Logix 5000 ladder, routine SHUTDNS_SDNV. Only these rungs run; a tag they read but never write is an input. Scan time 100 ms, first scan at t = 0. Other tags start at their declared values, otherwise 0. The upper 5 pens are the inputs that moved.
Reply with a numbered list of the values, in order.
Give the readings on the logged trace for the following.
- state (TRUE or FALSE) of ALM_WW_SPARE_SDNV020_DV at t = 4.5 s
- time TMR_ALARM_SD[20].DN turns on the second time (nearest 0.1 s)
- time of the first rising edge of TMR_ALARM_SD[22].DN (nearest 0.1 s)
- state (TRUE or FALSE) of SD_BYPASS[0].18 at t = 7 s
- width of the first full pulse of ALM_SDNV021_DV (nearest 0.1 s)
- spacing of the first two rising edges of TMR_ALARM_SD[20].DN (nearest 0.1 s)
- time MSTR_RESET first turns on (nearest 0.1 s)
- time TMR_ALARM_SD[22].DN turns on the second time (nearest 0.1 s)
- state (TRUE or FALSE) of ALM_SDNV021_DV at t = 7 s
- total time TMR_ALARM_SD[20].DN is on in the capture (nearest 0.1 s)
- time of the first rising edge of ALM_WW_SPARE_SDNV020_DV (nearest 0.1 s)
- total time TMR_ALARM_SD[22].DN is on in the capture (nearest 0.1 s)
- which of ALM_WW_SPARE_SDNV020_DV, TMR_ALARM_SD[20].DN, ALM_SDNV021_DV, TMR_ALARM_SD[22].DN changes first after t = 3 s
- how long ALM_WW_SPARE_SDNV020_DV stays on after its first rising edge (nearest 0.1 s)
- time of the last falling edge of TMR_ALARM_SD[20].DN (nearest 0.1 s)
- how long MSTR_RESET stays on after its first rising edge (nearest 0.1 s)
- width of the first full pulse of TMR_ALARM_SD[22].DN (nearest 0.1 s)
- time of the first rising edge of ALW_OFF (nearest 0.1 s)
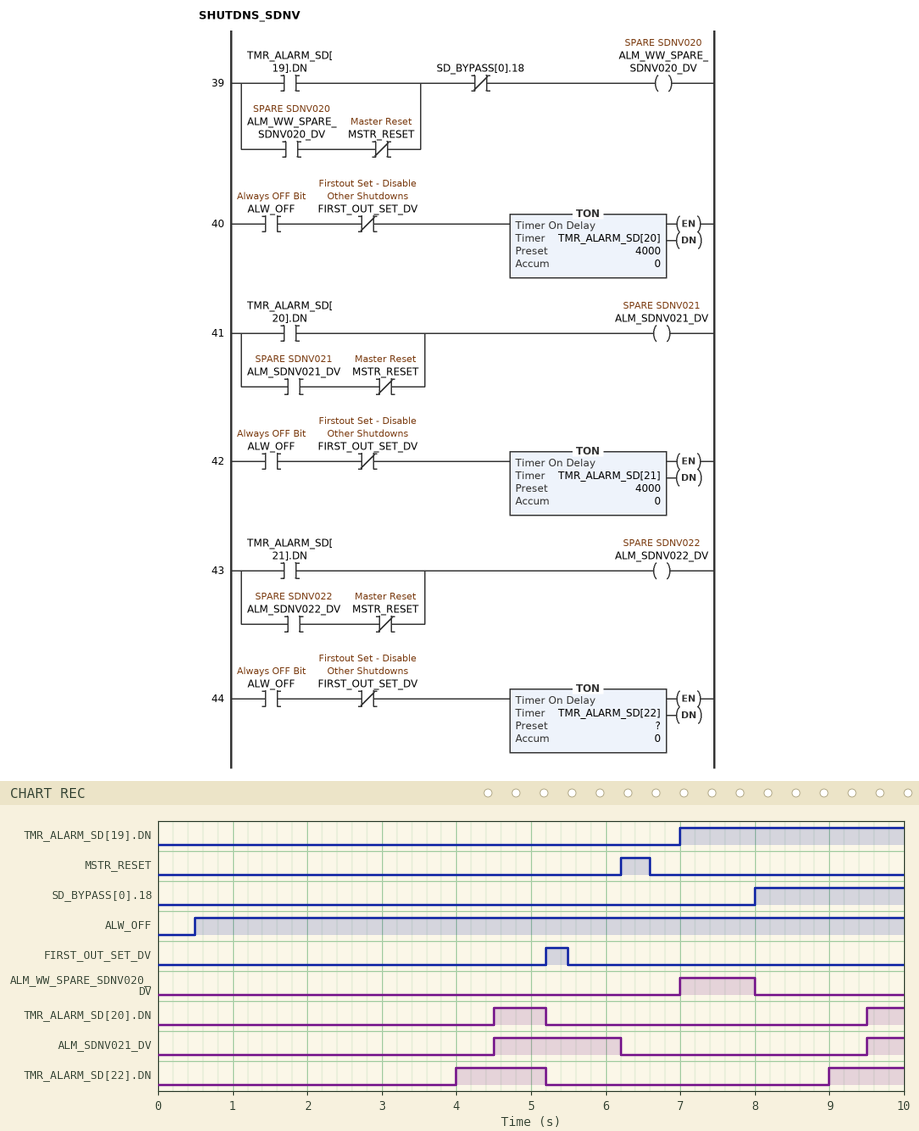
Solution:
1. FALSE
2. 9.5 s
3. 4.0 s
4. FALSE
5. 1.7 s
6. 5.0 s
7. 6.2 s
8. 9.0 s
9. FALSE
10. 1.2 s
11. 7.0 s
12. 2.2 s
13. TMR_ALARM_SD[22].DN
14. 1.0 s
15. 5.2 s
16. 0.4 s
17. 1.2 s
18. 0.5 s
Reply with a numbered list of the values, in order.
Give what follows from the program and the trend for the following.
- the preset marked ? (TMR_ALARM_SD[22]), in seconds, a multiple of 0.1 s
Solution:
1. 3.5 s
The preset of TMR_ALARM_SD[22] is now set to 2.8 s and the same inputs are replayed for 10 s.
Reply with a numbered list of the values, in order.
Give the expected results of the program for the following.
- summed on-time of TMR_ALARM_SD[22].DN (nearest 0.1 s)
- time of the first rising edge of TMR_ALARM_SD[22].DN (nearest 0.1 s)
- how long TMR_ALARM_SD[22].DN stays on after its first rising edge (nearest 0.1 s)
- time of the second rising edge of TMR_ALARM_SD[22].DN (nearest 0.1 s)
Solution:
1. 3.6 s
2. 3.3 s
3. 1.9 s
4. 8.3 s
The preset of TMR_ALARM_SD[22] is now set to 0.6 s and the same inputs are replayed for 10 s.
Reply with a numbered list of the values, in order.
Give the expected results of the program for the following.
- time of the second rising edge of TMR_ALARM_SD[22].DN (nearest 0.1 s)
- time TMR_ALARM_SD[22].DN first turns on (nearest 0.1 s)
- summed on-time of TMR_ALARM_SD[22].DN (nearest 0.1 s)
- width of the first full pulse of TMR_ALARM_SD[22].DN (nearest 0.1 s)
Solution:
1. 6.1 s
2. 1.1 s
3. 8.0 s
4. 4.1 s
